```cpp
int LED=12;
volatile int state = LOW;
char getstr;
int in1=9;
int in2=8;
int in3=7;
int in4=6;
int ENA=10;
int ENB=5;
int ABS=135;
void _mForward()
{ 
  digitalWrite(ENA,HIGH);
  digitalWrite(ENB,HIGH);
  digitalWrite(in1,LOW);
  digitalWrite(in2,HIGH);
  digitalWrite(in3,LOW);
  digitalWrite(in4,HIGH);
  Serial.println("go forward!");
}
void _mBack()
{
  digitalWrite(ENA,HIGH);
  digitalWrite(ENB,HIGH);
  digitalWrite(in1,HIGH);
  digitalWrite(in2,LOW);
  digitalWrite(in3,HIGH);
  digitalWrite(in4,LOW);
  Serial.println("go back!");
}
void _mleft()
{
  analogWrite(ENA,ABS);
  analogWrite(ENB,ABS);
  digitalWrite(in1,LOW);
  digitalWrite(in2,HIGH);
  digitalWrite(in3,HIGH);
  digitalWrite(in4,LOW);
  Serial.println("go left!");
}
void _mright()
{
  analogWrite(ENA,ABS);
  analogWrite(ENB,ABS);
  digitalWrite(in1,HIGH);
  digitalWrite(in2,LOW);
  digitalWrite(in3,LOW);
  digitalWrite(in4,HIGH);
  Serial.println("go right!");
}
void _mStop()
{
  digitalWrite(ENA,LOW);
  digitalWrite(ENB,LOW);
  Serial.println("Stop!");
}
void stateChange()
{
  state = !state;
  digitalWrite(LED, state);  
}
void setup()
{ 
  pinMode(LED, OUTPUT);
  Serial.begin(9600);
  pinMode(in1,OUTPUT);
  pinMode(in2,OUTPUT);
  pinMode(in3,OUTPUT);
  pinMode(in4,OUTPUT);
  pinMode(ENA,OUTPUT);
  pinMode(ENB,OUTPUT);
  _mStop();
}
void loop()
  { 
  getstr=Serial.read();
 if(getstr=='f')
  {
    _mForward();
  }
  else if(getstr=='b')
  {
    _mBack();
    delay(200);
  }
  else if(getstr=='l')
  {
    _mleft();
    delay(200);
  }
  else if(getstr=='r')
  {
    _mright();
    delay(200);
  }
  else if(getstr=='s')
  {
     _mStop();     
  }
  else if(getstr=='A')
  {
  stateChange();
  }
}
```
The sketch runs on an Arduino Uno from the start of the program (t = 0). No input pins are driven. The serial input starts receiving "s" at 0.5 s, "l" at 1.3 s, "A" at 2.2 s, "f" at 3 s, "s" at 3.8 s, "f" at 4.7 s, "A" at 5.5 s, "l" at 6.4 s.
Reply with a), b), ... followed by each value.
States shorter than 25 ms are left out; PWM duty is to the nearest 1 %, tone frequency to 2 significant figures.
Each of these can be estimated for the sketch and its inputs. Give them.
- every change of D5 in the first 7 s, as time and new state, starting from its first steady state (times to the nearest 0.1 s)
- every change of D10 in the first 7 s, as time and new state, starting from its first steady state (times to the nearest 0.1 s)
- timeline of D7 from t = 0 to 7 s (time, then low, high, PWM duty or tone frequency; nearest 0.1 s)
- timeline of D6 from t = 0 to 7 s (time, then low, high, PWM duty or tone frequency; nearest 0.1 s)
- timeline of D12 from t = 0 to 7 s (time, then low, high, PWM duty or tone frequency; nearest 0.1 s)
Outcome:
a) 0 s low; 1.3 s PWM 53 %; 3 s high; 3.8 s low; 4.7 s high; 6.4 s PWM 53 %
b) 0 s low; 1.3 s PWM 53 %; 3 s high; 3.8 s low; 4.7 s high; 6.4 s PWM 53 %
c) 0 s low; 1.3 s high; 3 s low; 6.4 s high
d) 0 s low; 3 s high; 6.4 s low
e) 0 s low; 2.2 s high; 5.5 s low
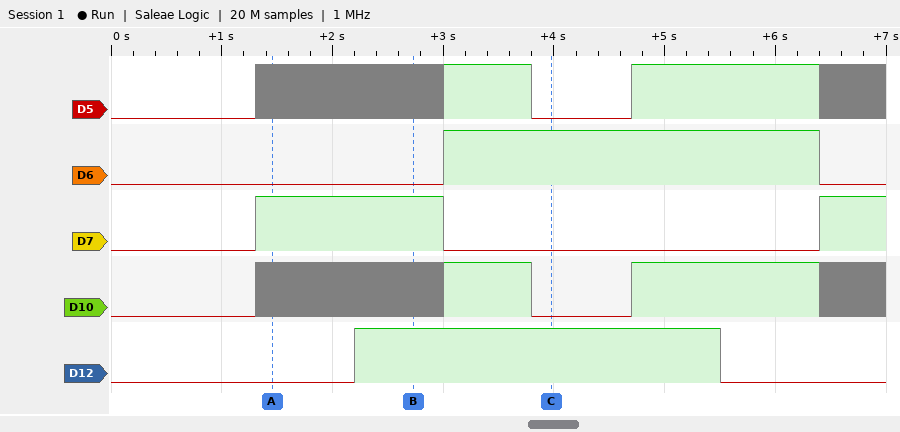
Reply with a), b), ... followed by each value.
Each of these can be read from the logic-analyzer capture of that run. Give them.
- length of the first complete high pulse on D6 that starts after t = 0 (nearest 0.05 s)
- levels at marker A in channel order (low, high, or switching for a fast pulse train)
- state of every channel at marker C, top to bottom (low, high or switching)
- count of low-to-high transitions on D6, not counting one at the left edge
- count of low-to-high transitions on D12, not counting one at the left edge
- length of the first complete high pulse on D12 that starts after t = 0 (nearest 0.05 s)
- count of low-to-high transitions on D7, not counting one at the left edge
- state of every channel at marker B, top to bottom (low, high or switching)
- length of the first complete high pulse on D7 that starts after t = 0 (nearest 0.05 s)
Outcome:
a) 3.40 s
b) D5 switching, D6 low, D7 high, D10 switching, D12 low
c) D5 low, D6 high, D7 low, D10 low, D12 high
d) 1
e) 1
f) 3.30 s
g) 2
h) D5 switching, D6 low, D7 high, D10 switching, D12 high
i) 1.70 s
